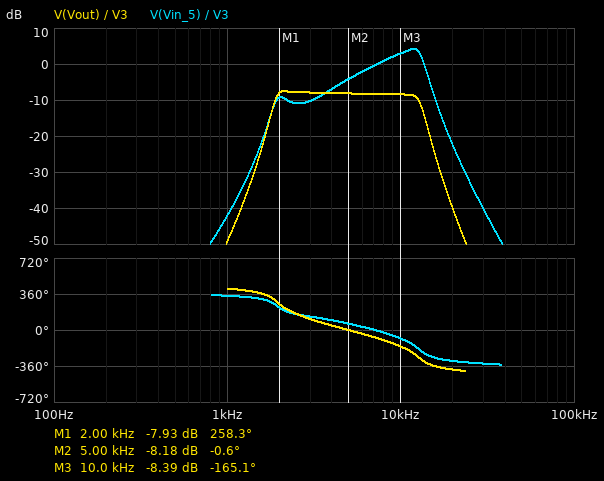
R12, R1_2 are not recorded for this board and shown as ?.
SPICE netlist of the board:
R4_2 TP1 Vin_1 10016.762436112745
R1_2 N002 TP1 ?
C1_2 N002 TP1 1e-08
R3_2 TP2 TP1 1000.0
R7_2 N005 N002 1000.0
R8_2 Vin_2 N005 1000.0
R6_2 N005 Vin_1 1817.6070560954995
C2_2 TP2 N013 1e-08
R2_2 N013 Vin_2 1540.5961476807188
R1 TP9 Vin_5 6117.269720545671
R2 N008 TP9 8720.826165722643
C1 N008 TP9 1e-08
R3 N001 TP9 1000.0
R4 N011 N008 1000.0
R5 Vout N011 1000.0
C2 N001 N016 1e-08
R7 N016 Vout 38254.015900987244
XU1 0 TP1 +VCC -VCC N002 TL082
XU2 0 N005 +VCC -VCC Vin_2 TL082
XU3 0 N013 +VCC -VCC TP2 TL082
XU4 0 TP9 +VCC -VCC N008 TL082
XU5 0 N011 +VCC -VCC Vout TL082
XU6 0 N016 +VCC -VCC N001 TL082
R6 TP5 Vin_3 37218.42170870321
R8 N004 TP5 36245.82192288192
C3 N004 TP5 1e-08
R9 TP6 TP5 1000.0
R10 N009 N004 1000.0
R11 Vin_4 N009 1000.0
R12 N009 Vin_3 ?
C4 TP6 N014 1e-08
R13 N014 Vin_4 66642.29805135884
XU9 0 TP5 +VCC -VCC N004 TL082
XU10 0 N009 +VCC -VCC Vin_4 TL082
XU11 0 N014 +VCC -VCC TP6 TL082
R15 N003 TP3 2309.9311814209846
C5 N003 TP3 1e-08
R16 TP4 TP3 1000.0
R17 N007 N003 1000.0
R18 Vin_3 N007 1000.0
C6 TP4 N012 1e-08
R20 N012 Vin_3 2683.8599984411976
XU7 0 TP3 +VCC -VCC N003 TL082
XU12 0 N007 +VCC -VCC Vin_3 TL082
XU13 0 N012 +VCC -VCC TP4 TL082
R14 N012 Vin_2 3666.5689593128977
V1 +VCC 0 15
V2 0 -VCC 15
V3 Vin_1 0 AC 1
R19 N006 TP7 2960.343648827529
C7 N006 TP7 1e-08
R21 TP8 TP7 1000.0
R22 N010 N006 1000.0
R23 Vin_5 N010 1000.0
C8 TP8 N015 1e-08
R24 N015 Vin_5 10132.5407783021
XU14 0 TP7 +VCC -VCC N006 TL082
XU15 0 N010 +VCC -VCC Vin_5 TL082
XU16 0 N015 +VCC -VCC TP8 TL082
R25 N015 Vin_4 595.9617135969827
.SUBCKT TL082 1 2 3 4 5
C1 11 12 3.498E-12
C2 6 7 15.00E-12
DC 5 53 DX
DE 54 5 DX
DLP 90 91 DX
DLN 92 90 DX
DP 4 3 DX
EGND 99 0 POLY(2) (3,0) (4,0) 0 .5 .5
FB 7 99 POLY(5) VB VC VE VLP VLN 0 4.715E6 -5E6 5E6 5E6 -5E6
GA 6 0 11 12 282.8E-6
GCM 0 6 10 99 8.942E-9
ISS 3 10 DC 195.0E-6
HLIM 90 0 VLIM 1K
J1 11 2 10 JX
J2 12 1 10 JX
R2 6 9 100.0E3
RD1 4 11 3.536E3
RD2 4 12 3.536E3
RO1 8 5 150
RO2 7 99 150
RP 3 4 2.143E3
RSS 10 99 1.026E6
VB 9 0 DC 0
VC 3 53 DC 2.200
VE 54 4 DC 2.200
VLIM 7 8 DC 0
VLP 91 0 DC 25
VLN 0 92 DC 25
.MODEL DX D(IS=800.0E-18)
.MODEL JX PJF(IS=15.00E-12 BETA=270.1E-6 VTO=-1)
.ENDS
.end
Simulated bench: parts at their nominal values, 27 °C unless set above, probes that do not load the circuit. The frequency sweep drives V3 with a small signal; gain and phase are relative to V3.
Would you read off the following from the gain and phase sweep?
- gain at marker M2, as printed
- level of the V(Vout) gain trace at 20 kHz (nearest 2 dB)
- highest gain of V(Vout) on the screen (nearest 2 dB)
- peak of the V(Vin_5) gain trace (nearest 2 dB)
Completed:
-8.18 dB
-40 dB
-8 dB
4 dB
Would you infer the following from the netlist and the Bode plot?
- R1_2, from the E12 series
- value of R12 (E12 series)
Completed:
4.7 kΩ
2.7 kΩ
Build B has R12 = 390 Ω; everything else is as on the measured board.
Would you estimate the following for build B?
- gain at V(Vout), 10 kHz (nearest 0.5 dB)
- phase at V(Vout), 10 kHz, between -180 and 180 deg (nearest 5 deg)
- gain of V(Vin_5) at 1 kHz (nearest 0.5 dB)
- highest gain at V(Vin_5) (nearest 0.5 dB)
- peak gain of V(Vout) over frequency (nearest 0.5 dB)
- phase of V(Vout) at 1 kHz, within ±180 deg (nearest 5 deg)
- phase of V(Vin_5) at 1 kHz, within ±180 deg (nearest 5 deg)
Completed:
8.5 dB
-170 deg
-27.0 dB
21.0 dB
9.0 dB
5 deg
-70 deg
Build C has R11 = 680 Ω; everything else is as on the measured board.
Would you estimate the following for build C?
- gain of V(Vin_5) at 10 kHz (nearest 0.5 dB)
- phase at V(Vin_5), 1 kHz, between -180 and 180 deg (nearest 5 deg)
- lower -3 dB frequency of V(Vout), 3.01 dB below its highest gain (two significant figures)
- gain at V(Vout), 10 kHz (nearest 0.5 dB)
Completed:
-0.5 dB
-25 deg
2.4 kHz
-12.0 dB
